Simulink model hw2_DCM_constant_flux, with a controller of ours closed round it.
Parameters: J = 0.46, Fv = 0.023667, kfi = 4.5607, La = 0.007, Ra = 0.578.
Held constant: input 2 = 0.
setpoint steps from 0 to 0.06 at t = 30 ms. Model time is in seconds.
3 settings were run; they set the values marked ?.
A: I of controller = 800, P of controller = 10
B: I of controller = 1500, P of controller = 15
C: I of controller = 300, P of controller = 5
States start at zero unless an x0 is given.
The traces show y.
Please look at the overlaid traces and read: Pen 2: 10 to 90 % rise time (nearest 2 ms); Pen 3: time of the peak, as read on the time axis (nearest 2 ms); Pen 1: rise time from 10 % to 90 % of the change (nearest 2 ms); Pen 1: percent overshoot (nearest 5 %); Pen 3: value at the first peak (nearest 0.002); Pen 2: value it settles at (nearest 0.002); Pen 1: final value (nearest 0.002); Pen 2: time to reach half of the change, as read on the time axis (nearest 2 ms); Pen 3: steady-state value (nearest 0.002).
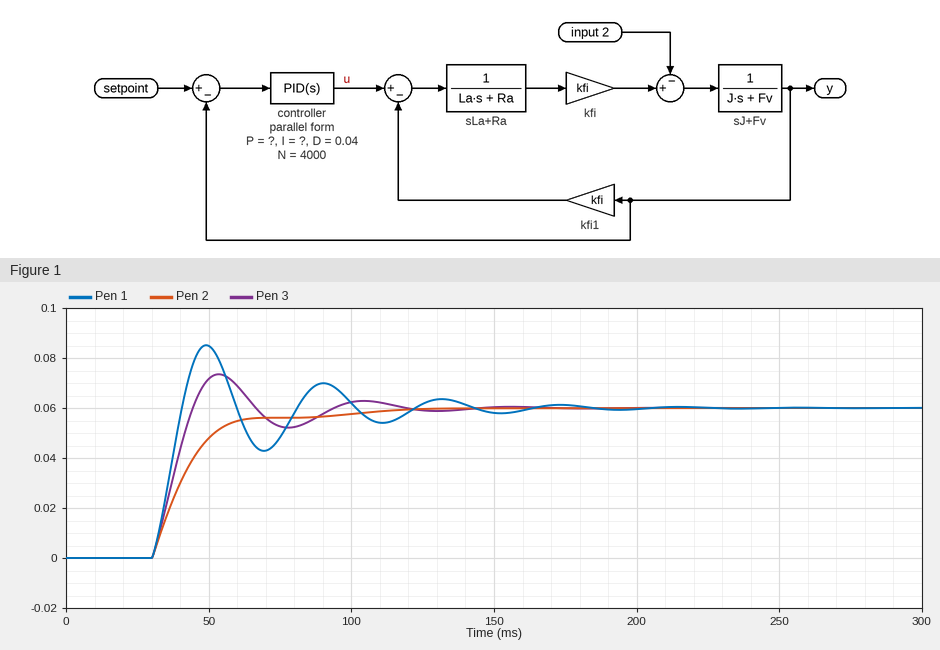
26 ms
54 ms
8 ms
40 %
0.074
0.060
0.060
40 ms
0.060
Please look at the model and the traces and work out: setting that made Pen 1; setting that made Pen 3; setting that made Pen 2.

B
A
C
